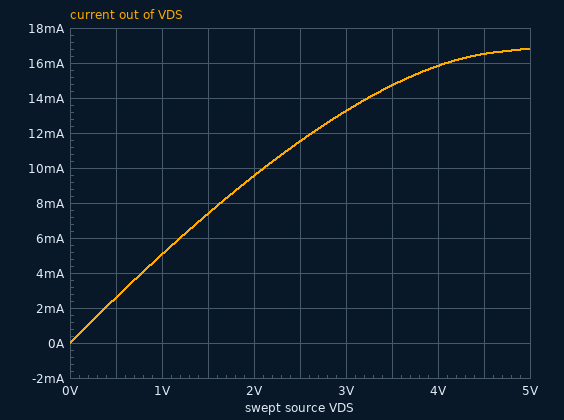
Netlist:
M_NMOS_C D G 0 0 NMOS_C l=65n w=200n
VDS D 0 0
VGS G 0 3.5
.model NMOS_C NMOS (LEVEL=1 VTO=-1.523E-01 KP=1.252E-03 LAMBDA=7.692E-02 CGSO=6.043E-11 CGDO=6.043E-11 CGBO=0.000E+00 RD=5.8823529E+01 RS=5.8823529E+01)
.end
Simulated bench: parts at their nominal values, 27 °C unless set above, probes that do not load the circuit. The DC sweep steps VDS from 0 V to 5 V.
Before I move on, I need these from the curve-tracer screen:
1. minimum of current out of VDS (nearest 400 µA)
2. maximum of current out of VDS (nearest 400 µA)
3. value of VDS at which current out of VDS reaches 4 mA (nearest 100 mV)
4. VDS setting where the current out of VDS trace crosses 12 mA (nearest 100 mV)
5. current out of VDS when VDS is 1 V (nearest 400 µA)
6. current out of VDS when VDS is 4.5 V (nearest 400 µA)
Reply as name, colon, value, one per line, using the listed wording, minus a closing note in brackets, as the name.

minimum of current out of VDS: 0 A
maximum of current out of VDS: 16.8 mA
value of VDS at which current out of VDS reaches 4 mA: 800 mV
VDS setting where the current out of VDS trace crosses 12 mA: 2.6 V
current out of VDS when VDS is 1 V: 5.2 mA
current out of VDS when VDS is 4.5 V: 16.4 mA
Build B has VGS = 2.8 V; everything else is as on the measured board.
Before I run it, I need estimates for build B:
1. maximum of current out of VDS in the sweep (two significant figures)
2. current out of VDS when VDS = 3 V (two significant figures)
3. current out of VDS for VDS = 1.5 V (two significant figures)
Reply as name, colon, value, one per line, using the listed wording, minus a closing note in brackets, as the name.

maximum of current out of VDS in the sweep: 12 mA
current out of VDS when VDS = 3 V: 11 mA
current out of VDS for VDS = 1.5 V: 6.5 mA
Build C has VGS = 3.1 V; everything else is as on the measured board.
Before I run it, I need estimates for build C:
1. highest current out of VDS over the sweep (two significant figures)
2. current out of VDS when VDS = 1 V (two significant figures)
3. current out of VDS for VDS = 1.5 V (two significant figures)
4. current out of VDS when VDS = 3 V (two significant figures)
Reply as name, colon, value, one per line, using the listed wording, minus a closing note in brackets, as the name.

highest current out of VDS over the sweep: 14 mA
current out of VDS when VDS = 1 V: 4.8 mA
current out of VDS for VDS = 1.5 V: 6.9 mA
current out of VDS when VDS = 3 V: 12 mA
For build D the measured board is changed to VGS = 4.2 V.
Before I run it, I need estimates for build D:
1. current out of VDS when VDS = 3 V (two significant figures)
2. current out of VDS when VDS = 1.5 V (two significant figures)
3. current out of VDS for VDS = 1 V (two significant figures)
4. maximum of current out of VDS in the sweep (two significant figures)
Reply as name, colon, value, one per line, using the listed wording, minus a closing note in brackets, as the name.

current out of VDS when VDS = 3 V: 15 mA
current out of VDS when VDS = 1.5 V: 8.0 mA
current out of VDS for VDS = 1 V: 5.5 mA
maximum of current out of VDS in the sweep: 21 mA
